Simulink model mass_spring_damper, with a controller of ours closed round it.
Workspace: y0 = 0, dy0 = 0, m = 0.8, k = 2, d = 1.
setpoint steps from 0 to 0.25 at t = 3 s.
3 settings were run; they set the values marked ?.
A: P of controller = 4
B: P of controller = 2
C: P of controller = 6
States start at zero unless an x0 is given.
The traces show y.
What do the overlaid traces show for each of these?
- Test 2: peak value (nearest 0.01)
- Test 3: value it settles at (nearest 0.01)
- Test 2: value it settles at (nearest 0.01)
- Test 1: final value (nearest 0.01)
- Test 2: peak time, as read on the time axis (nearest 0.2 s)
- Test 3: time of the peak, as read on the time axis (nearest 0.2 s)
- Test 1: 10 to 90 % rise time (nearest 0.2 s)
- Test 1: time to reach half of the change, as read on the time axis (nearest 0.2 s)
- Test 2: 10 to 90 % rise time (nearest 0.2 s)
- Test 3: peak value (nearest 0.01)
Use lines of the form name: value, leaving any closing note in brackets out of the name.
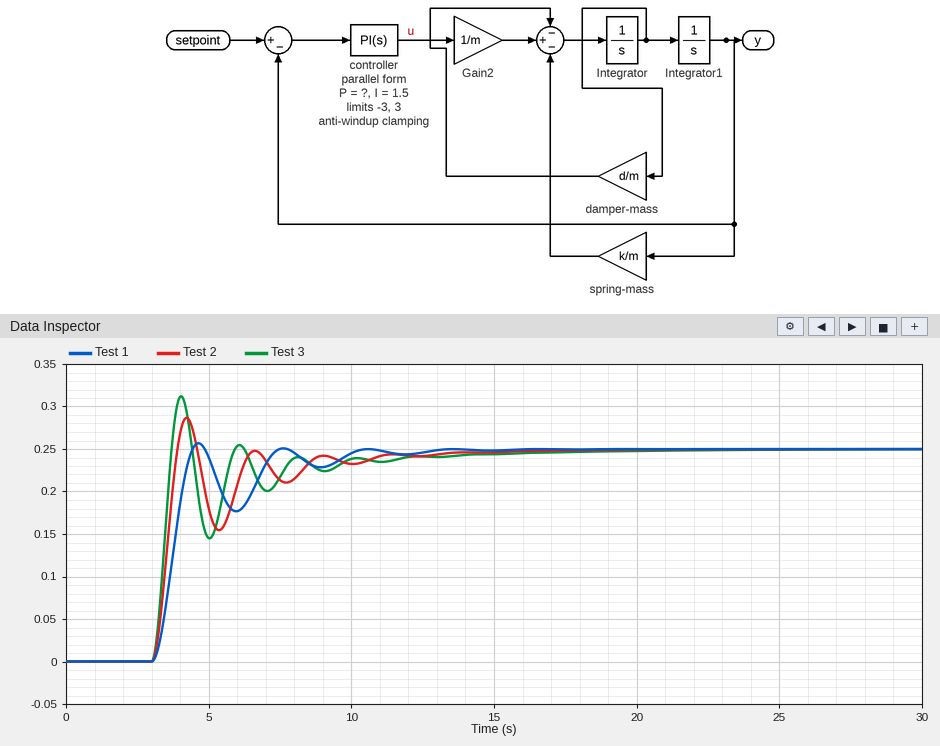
Test 2: peak value: 0.29
Test 3: value it settles at: 0.25
Test 2: value it settles at: 0.25
Test 1: final value: 0.25
Test 2: peak time, as read on the time axis: 4.2 s
Test 3: time of the peak, as read on the time axis: 4.0 s
Test 1: 10 to 90 % rise time: 1.0 s
Test 1: time to reach half of the change, as read on the time axis: 3.8 s
Test 2: 10 to 90 % rise time: 0.6 s
Test 3: peak value: 0.31
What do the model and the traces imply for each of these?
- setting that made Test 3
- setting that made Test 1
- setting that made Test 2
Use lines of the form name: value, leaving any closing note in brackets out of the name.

setting that made Test 3: C
setting that made Test 1: B
setting that made Test 2: A
